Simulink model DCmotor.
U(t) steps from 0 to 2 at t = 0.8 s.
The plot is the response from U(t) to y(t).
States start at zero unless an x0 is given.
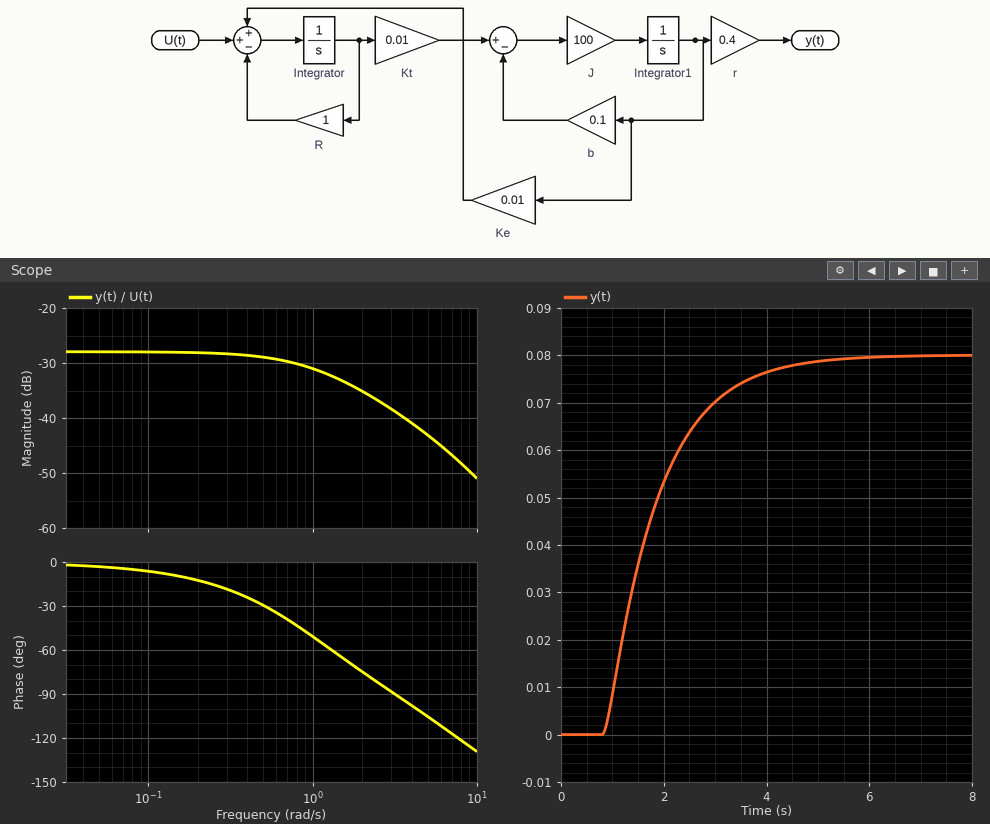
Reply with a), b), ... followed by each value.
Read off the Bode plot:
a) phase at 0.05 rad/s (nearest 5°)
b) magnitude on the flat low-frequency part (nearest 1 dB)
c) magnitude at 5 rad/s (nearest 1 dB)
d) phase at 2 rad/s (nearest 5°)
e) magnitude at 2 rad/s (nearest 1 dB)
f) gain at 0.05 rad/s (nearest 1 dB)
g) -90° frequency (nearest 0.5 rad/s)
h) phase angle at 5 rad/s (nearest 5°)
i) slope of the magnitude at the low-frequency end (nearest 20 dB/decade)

a) -5°
b) -28 dB
c) -43 dB
d) -75°
e) -35 dB
f) -28 dB
g) 3.0 rad/s
h) -105°
i) 0 dB/decade
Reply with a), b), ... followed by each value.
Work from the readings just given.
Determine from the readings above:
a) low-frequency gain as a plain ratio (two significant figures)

a) 0.040
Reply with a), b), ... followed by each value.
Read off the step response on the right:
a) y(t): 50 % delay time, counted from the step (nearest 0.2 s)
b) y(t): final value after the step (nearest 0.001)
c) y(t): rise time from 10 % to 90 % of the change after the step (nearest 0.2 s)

a) 0.8 s
b) 0.080
c) 2.2 s
